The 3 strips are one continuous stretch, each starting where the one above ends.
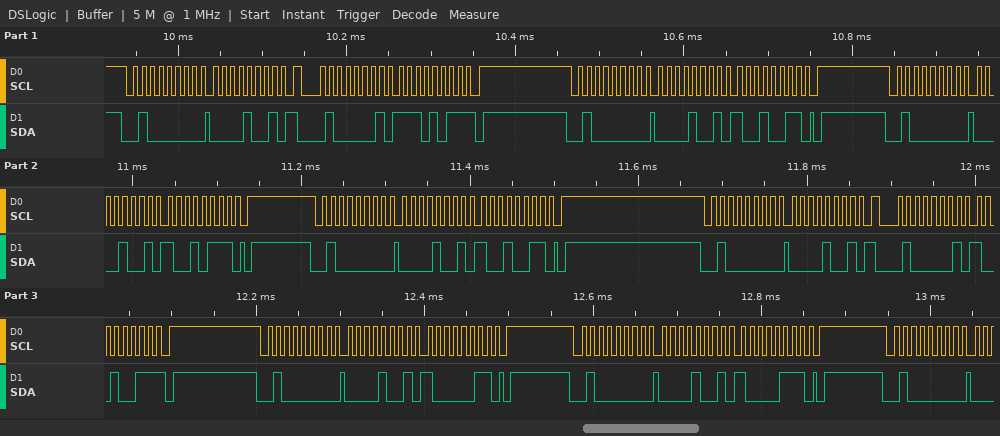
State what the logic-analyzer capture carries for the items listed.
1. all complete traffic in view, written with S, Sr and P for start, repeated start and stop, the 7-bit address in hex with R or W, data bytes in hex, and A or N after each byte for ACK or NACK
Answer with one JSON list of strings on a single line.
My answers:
["S 20W A 09 A Sr 20R A EB N P S 20W A 09 A 93 A P S 20W A 09 A 97 A P S 20W A 09 A 93 A P S 20W A 09 A Sr 20R A 93 N P S 20W A 09 A 83 A P S 20W A 09 A 87 A P S 20W A"]
